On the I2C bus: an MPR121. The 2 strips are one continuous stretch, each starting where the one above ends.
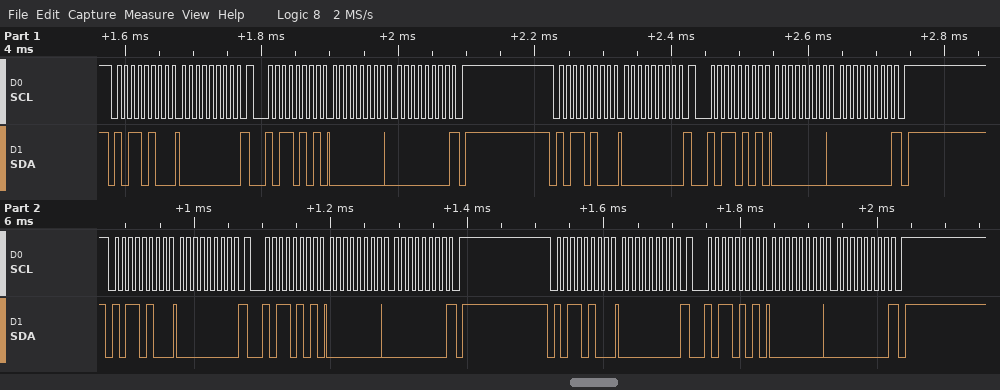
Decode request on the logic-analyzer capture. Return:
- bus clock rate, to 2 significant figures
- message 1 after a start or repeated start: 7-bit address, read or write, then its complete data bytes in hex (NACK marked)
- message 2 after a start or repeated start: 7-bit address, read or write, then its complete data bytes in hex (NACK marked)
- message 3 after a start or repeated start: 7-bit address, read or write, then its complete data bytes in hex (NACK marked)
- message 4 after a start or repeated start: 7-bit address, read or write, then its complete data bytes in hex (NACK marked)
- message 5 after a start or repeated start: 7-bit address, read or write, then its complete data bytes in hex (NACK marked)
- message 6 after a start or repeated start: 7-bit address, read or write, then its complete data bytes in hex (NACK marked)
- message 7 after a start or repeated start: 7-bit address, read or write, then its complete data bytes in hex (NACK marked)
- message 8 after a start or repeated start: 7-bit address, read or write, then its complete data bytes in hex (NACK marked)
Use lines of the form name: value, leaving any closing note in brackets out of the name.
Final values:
bus clock rate, to 2 significant figures: 100 kHz
message 1 after a start or repeated start: 7-bit address, read or write, then its complete data bytes in hex: 0x5A write: 00
message 2 after a start or repeated start: 7-bit address, read or write, then its complete data bytes in hex: 0x5A read: 00 00 NACK
message 3 after a start or repeated start: 7-bit address, read or write, then its complete data bytes in hex: 0x5A write: 00
message 4 after a start or repeated start: 7-bit address, read or write, then its complete data bytes in hex: 0x5A read: 00 00 NACK
message 5 after a start or repeated start: 7-bit address, read or write, then its complete data bytes in hex: 0x5A write: 00
message 6 after a start or repeated start: 7-bit address, read or write, then its complete data bytes in hex: 0x5A read: 00 00 NACK
message 7 after a start or repeated start: 7-bit address, read or write, then its complete data bytes in hex: 0x5A write: 00
message 8 after a start or repeated start: 7-bit address, read or write, then its complete data bytes in hex: 0x5A read: 00 00 NACK
